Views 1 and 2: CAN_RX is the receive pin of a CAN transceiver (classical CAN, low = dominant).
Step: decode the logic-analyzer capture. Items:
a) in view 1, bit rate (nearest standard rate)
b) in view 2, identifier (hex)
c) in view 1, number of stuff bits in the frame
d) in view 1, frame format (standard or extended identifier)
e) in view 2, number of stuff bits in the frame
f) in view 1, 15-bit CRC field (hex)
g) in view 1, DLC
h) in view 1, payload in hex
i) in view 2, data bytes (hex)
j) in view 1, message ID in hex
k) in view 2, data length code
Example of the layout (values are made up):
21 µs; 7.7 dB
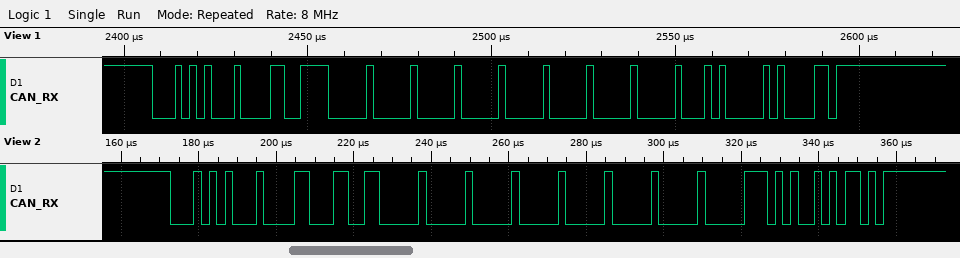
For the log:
500 kbit/s; 0x151; 9; standard; 8; 0x5021; 6; 78 00 00 00 00 00; 33 00 00 00 00 00; 0x151; 6
